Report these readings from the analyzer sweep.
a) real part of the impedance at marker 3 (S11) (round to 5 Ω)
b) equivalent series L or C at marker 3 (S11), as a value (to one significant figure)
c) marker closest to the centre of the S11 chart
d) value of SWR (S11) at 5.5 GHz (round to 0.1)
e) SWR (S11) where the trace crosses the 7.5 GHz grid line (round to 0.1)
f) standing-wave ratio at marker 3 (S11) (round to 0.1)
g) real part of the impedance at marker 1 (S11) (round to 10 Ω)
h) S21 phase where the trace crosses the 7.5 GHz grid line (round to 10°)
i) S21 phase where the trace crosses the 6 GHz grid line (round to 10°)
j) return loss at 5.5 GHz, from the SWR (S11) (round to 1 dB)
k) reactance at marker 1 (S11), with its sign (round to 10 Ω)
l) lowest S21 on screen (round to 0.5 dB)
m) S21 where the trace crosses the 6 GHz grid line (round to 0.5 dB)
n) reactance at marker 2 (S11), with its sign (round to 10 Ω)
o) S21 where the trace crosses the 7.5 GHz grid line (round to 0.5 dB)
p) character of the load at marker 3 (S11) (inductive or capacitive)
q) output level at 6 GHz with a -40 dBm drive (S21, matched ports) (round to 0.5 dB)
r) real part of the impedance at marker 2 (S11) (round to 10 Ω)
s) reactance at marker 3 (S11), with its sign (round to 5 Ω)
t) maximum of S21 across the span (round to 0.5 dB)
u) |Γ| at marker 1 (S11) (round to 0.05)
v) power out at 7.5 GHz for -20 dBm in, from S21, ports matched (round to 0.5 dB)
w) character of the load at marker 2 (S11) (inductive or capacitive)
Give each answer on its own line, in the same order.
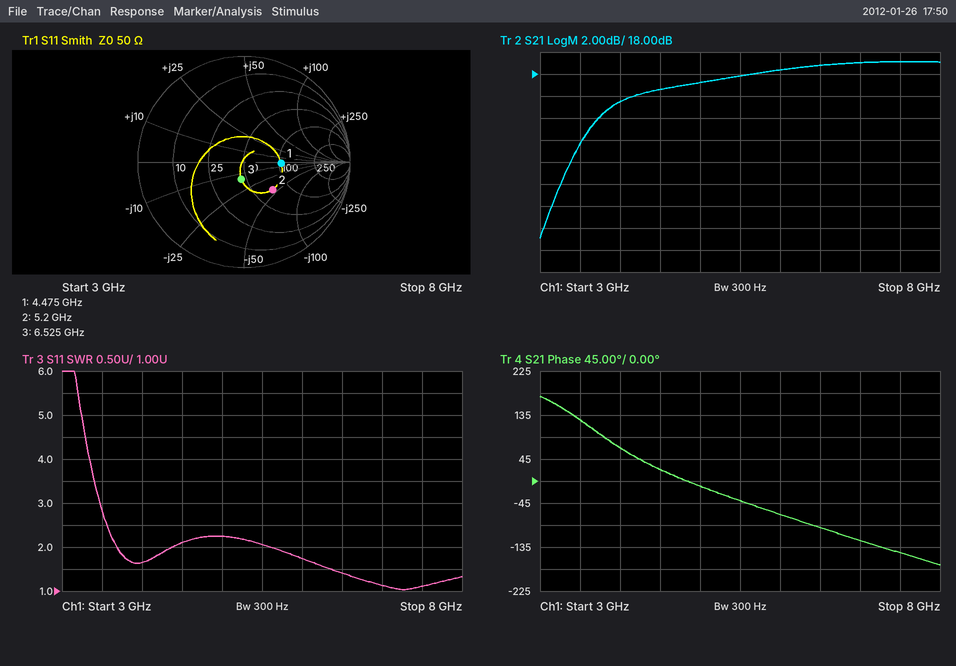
45 Ω
2 pF
marker 3
2.1
1.1
1.4
100 Ω
-150°
-70°
9 dB
0 Ω
3.0 dB
18.5 dB
-40 Ω
19.0 dB
capacitive
-21.5 dBm
70 Ω
-15 Ω
19.0 dB
0.35
-1.0 dBm
capacitive
